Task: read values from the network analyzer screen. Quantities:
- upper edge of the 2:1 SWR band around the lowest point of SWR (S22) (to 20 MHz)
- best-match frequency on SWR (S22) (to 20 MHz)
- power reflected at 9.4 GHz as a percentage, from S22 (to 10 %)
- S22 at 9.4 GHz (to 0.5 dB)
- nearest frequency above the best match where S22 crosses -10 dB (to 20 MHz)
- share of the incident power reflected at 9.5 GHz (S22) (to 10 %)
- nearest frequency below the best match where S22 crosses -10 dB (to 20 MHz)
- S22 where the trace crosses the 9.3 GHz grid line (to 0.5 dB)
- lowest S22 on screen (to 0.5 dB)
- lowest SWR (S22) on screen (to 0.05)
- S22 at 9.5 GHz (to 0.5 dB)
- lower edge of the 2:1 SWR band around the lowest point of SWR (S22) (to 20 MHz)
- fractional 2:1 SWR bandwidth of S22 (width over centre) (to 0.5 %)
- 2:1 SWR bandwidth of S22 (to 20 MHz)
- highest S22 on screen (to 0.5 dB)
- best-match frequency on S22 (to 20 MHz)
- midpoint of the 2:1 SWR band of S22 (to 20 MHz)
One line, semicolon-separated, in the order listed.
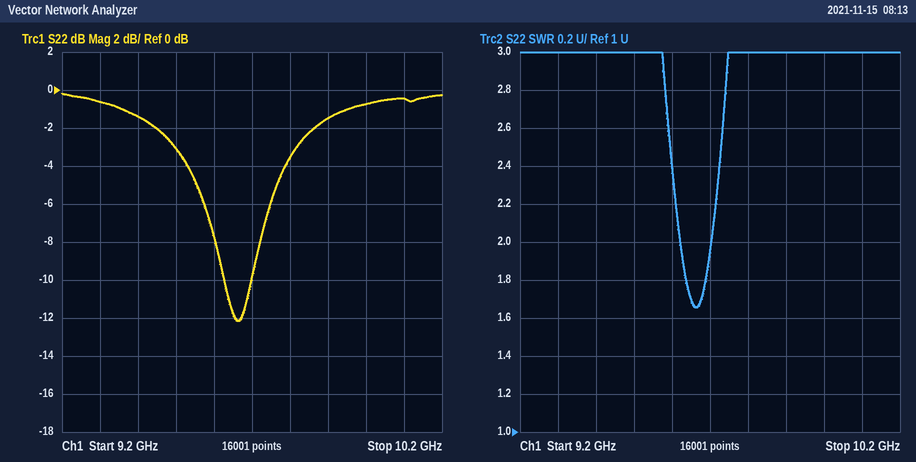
9.70 GHz; 9.66 GHz; 70 %; -1.5 dB; 9.70 GHz; 50 %; 9.62 GHz; -0.5 dB; -12.0 dB; 1.65; -3.0 dB; 9.62 GHz; 1.0 %; 80 MHz; 0.0 dB; 9.66 GHz; 9.66 GHz
